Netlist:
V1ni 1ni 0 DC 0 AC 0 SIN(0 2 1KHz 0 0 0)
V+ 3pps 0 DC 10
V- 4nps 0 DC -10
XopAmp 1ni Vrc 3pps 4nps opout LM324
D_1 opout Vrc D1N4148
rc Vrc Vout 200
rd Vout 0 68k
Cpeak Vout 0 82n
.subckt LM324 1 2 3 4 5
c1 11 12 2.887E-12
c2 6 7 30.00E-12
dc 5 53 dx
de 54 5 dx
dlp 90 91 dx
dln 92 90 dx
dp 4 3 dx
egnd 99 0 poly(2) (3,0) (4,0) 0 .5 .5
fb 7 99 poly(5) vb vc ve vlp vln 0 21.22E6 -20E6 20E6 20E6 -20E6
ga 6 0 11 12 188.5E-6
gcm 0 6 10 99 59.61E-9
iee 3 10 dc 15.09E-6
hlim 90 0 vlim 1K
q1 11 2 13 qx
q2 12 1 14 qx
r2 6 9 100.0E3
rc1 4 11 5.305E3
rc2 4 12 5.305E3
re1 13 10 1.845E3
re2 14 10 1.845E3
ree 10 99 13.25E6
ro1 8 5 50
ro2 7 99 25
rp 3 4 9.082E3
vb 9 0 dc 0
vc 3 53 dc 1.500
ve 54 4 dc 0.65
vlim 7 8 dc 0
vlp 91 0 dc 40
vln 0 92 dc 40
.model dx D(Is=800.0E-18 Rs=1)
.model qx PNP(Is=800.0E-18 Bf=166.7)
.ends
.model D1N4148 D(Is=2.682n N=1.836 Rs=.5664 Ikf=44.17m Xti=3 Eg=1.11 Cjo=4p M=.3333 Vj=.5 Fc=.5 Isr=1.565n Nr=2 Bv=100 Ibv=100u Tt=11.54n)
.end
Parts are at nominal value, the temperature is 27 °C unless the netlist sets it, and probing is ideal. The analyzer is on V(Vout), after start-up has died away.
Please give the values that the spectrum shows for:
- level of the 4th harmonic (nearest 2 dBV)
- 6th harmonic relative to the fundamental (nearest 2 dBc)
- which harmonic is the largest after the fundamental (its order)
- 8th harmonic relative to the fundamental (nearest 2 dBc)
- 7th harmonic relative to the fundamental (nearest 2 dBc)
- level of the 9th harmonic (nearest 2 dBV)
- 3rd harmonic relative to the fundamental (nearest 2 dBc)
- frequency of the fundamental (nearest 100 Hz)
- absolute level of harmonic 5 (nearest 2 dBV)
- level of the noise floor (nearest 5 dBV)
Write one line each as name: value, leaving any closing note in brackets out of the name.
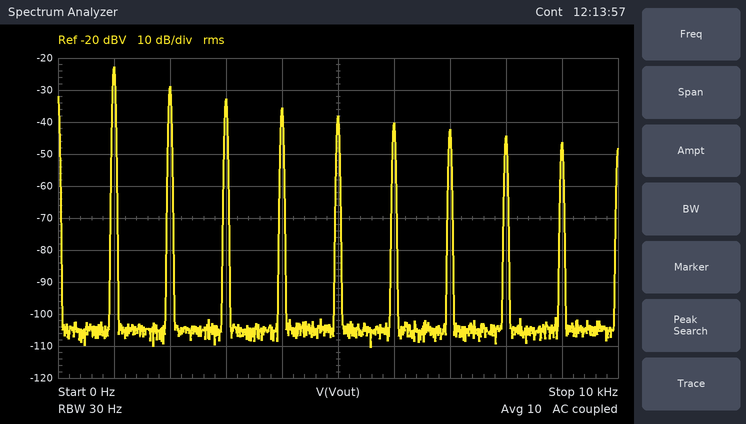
level of the 4th harmonic: -36 dBV
6th harmonic relative to the fundamental: -18 dBc
which harmonic is the largest after the fundamental: 2
8th harmonic relative to the fundamental: -22 dBc
7th harmonic relative to the fundamental: -20 dBc
level of the 9th harmonic: -46 dBV
3rd harmonic relative to the fundamental: -10 dBc
frequency of the fundamental: 1.0 kHz
absolute level of harmonic 5: -38 dBV
level of the noise floor: -105 dBV
